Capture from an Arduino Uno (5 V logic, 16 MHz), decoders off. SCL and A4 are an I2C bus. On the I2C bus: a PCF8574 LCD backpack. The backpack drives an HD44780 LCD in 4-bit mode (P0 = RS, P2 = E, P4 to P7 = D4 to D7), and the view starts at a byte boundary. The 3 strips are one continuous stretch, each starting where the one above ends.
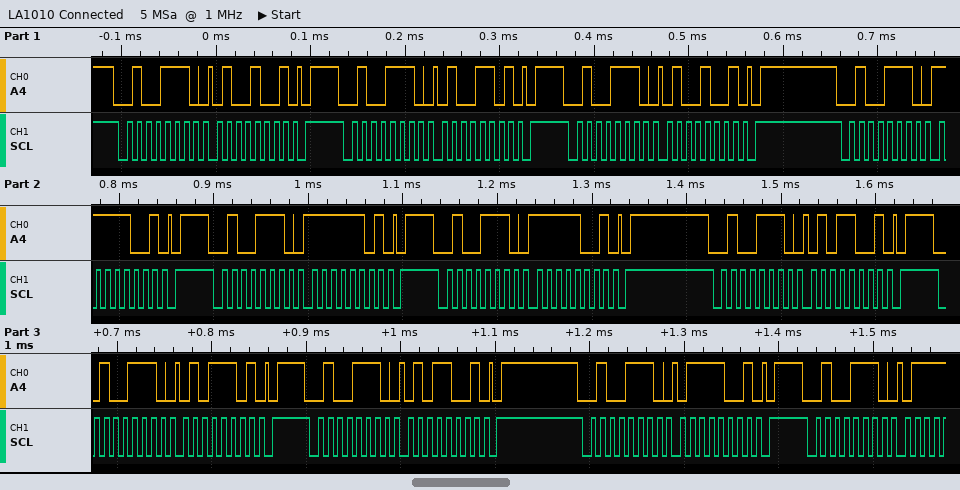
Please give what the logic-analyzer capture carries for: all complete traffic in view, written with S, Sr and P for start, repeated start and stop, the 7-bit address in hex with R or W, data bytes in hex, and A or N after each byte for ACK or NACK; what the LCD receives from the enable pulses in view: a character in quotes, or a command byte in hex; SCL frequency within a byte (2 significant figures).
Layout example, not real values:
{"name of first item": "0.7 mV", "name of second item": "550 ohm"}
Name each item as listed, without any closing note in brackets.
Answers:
{"all complete traffic in view, written with S, Sr and P for start, repeated start and stop, the 7-bit address in hex with R or W, data bytes in hex, and A or N after each byte for ACK or NACK": "S 27W A 49 A P S 27W A 4D A P S 27W A 49 A P S 27W A F9 A P S 27W A FD A P S 27W A F9 A P S 27W A 59 A P S 27W A 5D A P S 27W A 59 A P S 27W A 79 A P S 27W A", "what the LCD receives from the enable pulses in view: a character in quotes, or a command byte in hex": "'O'", "SCL frequency within a byte": "100 kHz"}
